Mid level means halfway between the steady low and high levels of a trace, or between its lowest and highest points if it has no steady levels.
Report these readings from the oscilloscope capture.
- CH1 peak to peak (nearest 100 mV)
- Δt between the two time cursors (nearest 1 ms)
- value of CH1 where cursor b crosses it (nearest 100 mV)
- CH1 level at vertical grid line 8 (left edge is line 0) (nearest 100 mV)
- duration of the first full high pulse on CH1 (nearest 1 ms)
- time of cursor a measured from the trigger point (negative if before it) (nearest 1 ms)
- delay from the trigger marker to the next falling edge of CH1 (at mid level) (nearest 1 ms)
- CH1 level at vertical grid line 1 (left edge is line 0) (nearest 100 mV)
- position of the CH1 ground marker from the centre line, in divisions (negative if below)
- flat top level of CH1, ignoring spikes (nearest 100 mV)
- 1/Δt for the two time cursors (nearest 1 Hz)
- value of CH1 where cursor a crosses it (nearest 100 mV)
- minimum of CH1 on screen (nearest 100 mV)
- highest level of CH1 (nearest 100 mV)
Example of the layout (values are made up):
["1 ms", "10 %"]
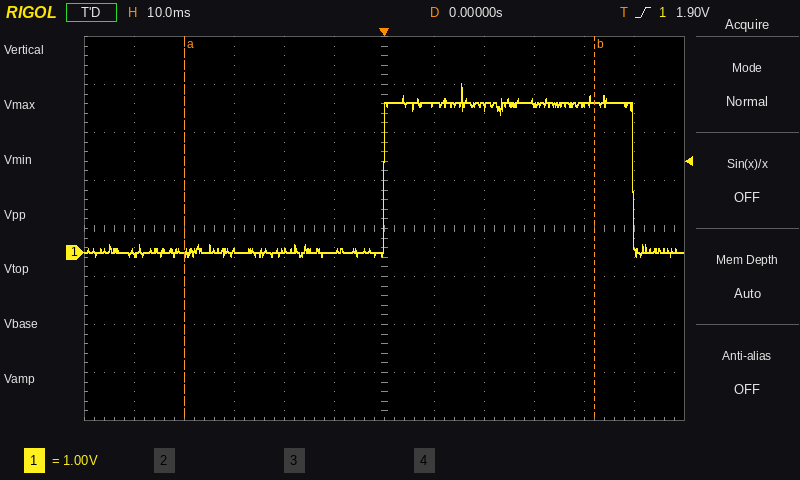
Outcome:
["3.6 V", "82 ms", "3.1 V", "3.0 V", "50 ms", "-40 ms", "50 ms", "0.0 V", "-0.5 div", "3.1 V", "12 Hz", "0.0 V", "-100 mV", "3.5 V"]
